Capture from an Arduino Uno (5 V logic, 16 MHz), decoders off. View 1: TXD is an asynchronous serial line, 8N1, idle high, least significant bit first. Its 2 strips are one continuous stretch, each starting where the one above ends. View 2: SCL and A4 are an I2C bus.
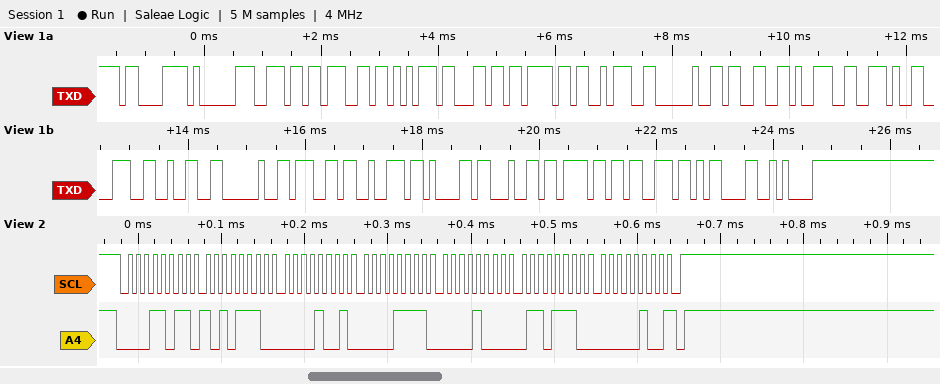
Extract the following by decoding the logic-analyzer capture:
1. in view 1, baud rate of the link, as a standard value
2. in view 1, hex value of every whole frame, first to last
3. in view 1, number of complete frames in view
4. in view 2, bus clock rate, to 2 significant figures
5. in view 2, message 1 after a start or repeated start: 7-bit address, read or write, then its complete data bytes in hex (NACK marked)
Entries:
9600 baud
C3 81 6E 67 75 6C 6F 3A 20 33 39 2E 38 32 20 67 72 61 64 6F 73 0D 0A
23
100 kHz
0x0D read: AE 09 0F 08 6E 04 NACK
